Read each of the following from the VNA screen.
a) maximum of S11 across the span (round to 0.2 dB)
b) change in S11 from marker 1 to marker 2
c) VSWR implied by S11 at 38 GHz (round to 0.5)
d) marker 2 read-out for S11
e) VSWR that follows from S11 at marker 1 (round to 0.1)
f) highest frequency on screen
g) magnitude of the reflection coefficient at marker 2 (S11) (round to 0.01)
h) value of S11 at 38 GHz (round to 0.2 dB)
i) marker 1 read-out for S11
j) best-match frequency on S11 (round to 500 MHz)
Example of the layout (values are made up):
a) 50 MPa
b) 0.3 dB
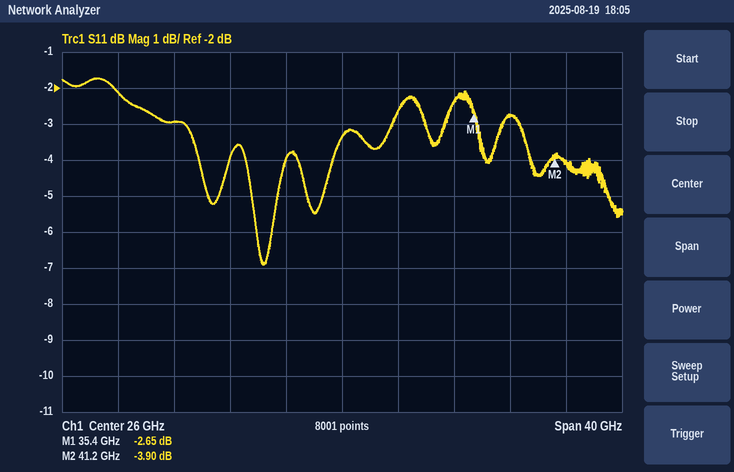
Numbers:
a) -1.8 dB
b) -1.25 dB
c) 6.5
d) -3.90 dB
e) 6.6
f) 46 GHz
g) 0.64
h) -2.8 dB
i) -2.65 dB
j) 20.5 GHz
